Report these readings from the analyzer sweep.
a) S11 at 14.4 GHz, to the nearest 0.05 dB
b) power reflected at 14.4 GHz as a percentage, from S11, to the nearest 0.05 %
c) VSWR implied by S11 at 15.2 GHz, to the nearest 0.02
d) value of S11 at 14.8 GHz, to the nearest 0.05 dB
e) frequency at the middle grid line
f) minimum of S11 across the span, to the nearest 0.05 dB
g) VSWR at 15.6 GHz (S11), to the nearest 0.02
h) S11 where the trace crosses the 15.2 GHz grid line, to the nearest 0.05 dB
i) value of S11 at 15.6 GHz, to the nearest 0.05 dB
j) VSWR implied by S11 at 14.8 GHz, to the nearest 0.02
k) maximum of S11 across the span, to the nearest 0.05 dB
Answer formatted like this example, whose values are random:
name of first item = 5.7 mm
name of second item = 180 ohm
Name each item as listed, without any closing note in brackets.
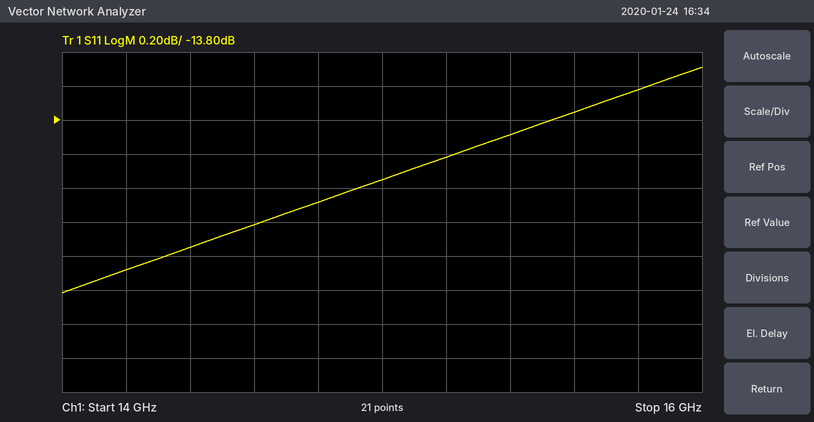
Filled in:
S11 at 14.4 GHz, to the nearest 0.05 dB = -14.55 dB
power reflected at 14.4 GHz as a percentage, from S11, to the nearest 0.05 % = 3.50 %
VSWR implied by S11 at 15.2 GHz, to the nearest 0.02 = 1.50
value of S11 at 14.8 GHz, to the nearest 0.05 dB = -14.30 dB
frequency at the middle grid line = 15 GHz
minimum of S11 across the span, to the nearest 0.05 dB = -14.80 dB
VSWR at 15.6 GHz (S11), to the nearest 0.02 = 1.52
S11 where the trace crosses the 15.2 GHz grid line, to the nearest 0.05 dB = -14.00 dB
value of S11 at 15.6 GHz, to the nearest 0.05 dB = -13.75 dB
VSWR implied by S11 at 14.8 GHz, to the nearest 0.02 = 1.48
maximum of S11 across the span, to the nearest 0.05 dB = -13.50 dB
